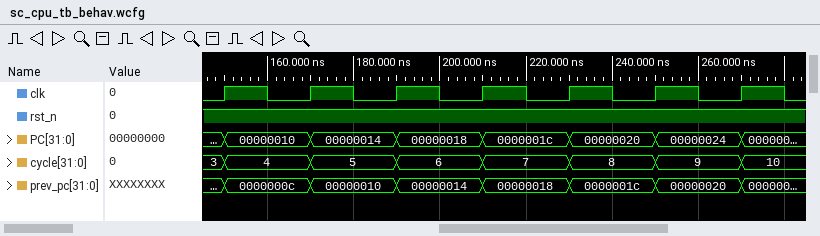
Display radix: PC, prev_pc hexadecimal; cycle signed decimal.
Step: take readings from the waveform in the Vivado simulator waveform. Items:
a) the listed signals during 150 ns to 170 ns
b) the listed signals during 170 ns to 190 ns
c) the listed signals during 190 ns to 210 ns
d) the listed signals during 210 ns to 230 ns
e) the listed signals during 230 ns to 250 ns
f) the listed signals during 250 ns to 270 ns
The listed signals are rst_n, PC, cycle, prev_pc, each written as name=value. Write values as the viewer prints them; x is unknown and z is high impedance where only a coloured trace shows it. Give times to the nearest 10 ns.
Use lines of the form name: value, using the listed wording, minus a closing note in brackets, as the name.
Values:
the listed signals during 150 ns to 170 ns: rst_n=1, PC=00000010, cycle=4, prev_pc=0000000c
the listed signals during 170 ns to 190 ns: rst_n=1, PC=00000014, cycle=5, prev_pc=00000010
the listed signals during 190 ns to 210 ns: rst_n=1, PC=00000018, cycle=6, prev_pc=00000014
the listed signals during 210 ns to 230 ns: rst_n=1, PC=0000001c, cycle=7, prev_pc=00000018
the listed signals during 230 ns to 250 ns: rst_n=1, PC=00000020, cycle=8, prev_pc=0000001c
the listed signals during 250 ns to 270 ns: rst_n=1, PC=00000024, cycle=9, prev_pc=00000020
